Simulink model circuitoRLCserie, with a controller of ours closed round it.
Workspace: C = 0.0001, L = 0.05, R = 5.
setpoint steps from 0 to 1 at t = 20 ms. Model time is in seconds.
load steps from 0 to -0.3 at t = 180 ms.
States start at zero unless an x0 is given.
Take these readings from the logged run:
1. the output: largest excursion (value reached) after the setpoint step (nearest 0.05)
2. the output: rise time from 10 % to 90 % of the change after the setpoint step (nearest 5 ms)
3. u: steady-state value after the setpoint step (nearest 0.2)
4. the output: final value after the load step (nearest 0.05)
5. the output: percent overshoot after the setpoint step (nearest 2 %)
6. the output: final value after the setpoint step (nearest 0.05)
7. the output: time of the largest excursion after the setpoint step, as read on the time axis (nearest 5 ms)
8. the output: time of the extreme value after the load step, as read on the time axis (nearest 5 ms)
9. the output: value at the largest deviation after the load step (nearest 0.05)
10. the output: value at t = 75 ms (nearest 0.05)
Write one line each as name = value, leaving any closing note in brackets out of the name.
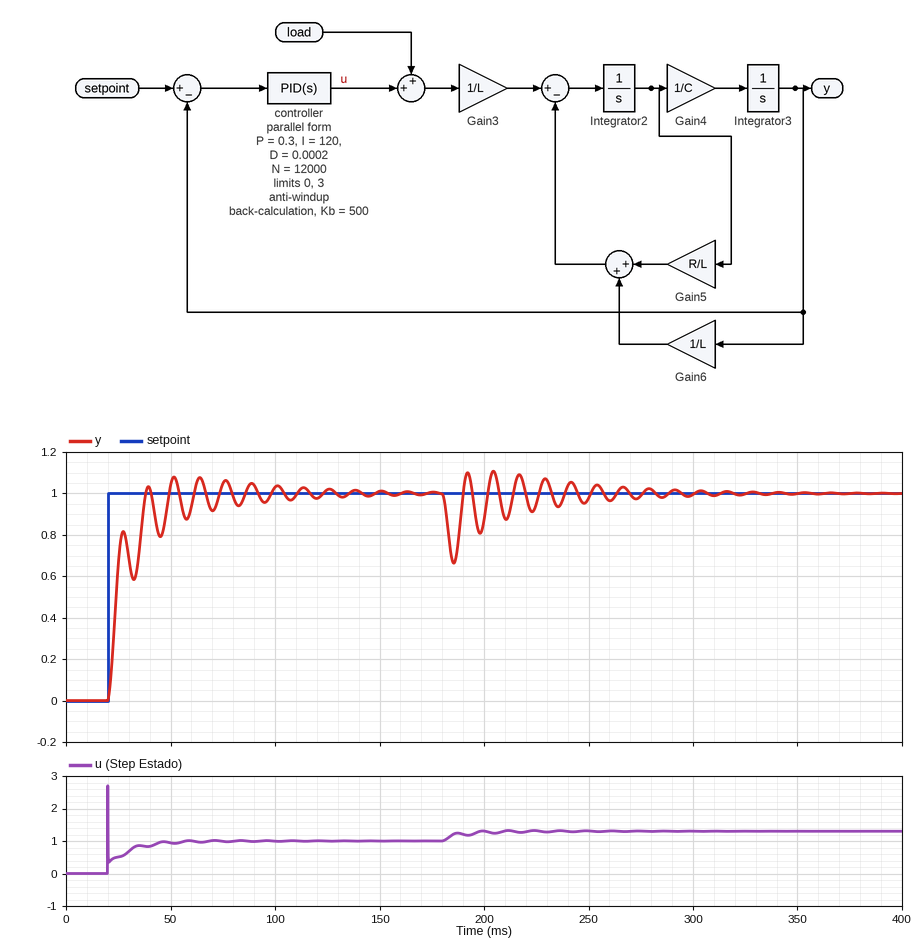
the output: largest excursion (value reached) after the setpoint step = 1.10
the output: rise time from 10 % to 90 % of the change after the setpoint step = 15 ms
u: steady-state value after the setpoint step = 1.0
the output: final value after the load step = 1.00
the output: percent overshoot after the setpoint step = 8 %
the output: final value after the setpoint step = 1.00
the output: time of the largest excursion after the setpoint step, as read on the time axis = 50 ms
the output: time of the extreme value after the load step, as read on the time axis = 185 ms
the output: value at the largest deviation after the load step = 0.65
the output: value at t = 75 ms = 1.05
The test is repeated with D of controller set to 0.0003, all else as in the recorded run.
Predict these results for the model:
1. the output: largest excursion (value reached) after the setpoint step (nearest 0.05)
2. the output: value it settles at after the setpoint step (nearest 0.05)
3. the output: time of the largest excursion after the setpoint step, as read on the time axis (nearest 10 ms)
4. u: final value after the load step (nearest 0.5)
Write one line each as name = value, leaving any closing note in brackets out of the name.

the output: largest excursion (value reached) after the setpoint step = 1.05
the output: value it settles at after the setpoint step = 1.00
the output: time of the largest excursion after the setpoint step, as read on the time axis = 60 ms
u: final value after the load step = 1.5
